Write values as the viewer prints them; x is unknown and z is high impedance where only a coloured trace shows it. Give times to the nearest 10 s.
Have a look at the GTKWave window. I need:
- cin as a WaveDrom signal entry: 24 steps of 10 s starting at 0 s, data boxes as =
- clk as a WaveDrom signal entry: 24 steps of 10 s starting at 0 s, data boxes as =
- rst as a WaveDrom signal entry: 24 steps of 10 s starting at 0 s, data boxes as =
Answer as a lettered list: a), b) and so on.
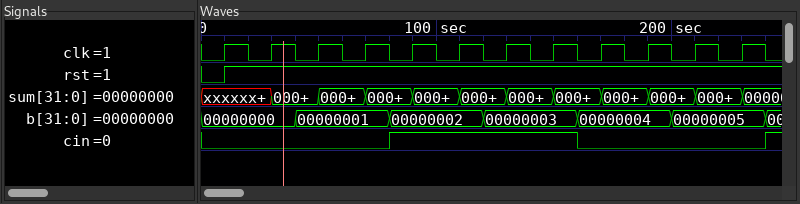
a) {name: 'cin', wave: '0.......1.......0.......'}
b) {name: 'clk', wave: '010101010101010101010101'}
c) {name: 'rst', wave: '01......................'}
